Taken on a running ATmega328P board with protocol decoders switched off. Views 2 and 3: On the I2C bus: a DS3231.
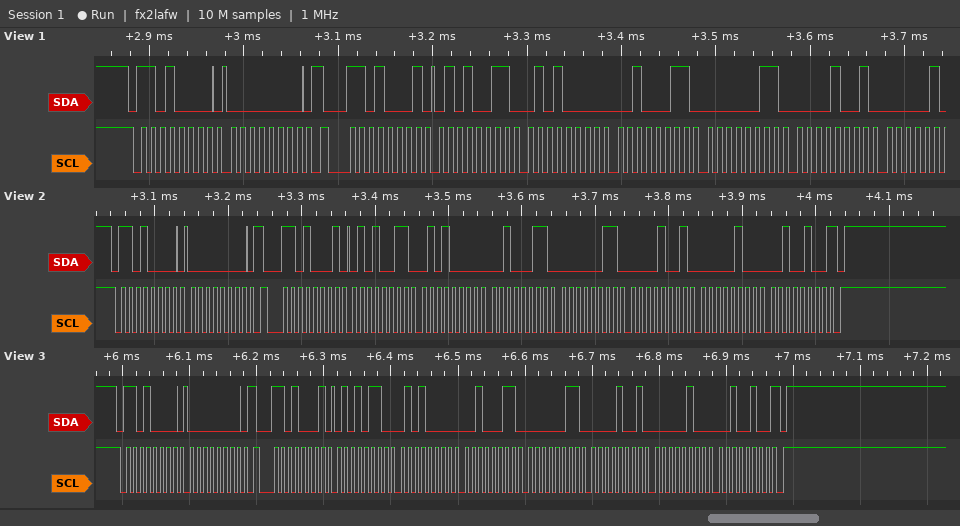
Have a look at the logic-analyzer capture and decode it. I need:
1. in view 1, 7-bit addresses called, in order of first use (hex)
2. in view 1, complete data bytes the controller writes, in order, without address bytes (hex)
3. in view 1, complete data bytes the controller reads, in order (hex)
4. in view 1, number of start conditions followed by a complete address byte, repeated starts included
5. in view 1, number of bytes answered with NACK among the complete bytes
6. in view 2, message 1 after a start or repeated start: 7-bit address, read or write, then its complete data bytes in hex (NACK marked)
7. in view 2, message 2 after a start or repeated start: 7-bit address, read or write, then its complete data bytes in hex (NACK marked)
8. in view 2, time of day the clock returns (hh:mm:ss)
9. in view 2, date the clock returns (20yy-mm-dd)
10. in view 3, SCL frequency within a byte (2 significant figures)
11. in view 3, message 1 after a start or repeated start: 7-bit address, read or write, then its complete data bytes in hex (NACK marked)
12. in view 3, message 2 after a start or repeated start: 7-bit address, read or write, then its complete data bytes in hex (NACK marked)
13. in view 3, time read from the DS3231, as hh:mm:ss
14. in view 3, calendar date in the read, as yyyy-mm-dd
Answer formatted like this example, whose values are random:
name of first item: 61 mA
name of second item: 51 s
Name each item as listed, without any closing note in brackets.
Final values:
in view 1, 7-bit addresses called, in order of first use: 0x68
in view 1, complete data bytes the controller writes, in order, without address bytes: 00
in view 1, complete data bytes the controller reads, in order: 53 50 23 03 09
in view 1, number of start conditions followed by a complete address byte, repeated starts included: 2
in view 1, number of bytes answered with NACK among the complete bytes: 0
in view 2, message 1 after a start or repeated start: 7-bit address, read or write, then its complete data bytes in hex: 0x68 write: 00
in view 2, message 2 after a start or repeated start: 7-bit address, read or write, then its complete data bytes in hex: 0x68 read: 53 50 23 03 09 04 24 NACK
in view 2, time of day the clock returns: 23:50:53
in view 2, date the clock returns: 2024-04-09
in view 3, SCL frequency within a byte: 100 kHz
in view 3, message 1 after a start or repeated start: 7-bit address, read or write, then its complete data bytes in hex: 0x68 write: 00
in view 3, message 2 after a start or repeated start: 7-bit address, read or write, then its complete data bytes in hex: 0x68 read: 56 50 23 03 09 04 24 NACK
in view 3, time read from the DS3231, as hh:mm:ss: 23:50:56
in view 3, calendar date in the read, as yyyy-mm-dd: 2024-04-09
